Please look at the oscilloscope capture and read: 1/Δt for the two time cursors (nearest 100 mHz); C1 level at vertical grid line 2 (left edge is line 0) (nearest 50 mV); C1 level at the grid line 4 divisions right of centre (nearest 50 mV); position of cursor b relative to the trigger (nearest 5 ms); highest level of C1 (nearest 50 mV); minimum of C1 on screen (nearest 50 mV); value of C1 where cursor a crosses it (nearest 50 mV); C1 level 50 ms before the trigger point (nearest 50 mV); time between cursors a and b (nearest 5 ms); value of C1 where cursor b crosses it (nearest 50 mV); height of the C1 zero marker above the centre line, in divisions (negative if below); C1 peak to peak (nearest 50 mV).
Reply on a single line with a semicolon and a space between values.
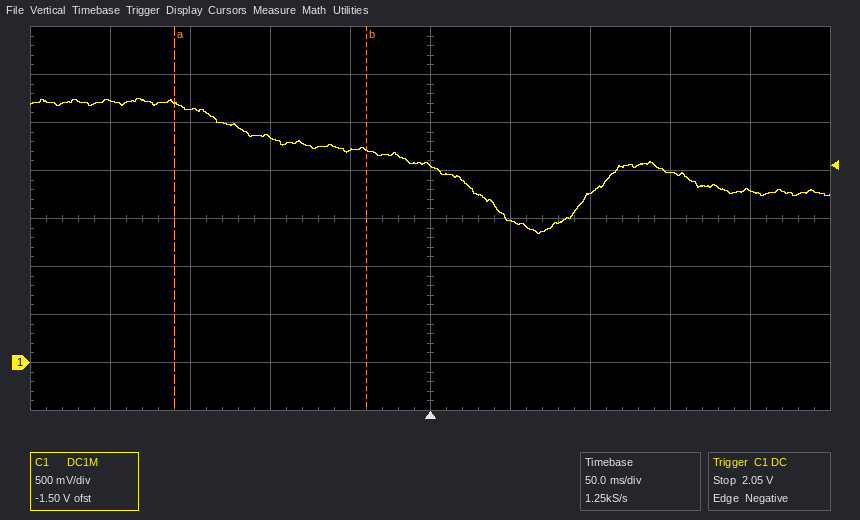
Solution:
8.3 Hz; 2.65 V; 1.80 V; -40 ms; 2.75 V; 1.35 V; 2.70 V; 2.20 V; 120 ms; 2.20 V; -3.0 div; 1.40 V
